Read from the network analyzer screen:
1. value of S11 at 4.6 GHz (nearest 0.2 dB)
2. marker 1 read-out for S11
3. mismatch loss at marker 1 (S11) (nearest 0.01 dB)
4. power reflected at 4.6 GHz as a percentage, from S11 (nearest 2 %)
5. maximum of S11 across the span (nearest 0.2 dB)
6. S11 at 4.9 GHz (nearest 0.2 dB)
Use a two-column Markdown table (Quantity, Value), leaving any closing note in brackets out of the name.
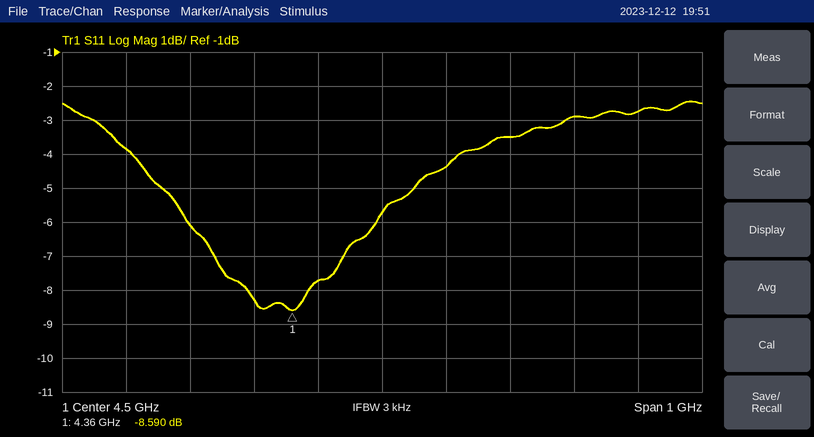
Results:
| Quantity | Value |
|---|---|
| value of S11 at 4.6 GHz | -4.4 dB |
| marker 1 read-out for S11 | -8.590 dB |
| mismatch loss at marker 1 (S11) | 0.65 dB |
| power reflected at 4.6 GHz as a percentage, from S11 | 36 % |
| maximum of S11 across the span | -2.4 dB |
| S11 at 4.9 GHz | -2.8 dB |
